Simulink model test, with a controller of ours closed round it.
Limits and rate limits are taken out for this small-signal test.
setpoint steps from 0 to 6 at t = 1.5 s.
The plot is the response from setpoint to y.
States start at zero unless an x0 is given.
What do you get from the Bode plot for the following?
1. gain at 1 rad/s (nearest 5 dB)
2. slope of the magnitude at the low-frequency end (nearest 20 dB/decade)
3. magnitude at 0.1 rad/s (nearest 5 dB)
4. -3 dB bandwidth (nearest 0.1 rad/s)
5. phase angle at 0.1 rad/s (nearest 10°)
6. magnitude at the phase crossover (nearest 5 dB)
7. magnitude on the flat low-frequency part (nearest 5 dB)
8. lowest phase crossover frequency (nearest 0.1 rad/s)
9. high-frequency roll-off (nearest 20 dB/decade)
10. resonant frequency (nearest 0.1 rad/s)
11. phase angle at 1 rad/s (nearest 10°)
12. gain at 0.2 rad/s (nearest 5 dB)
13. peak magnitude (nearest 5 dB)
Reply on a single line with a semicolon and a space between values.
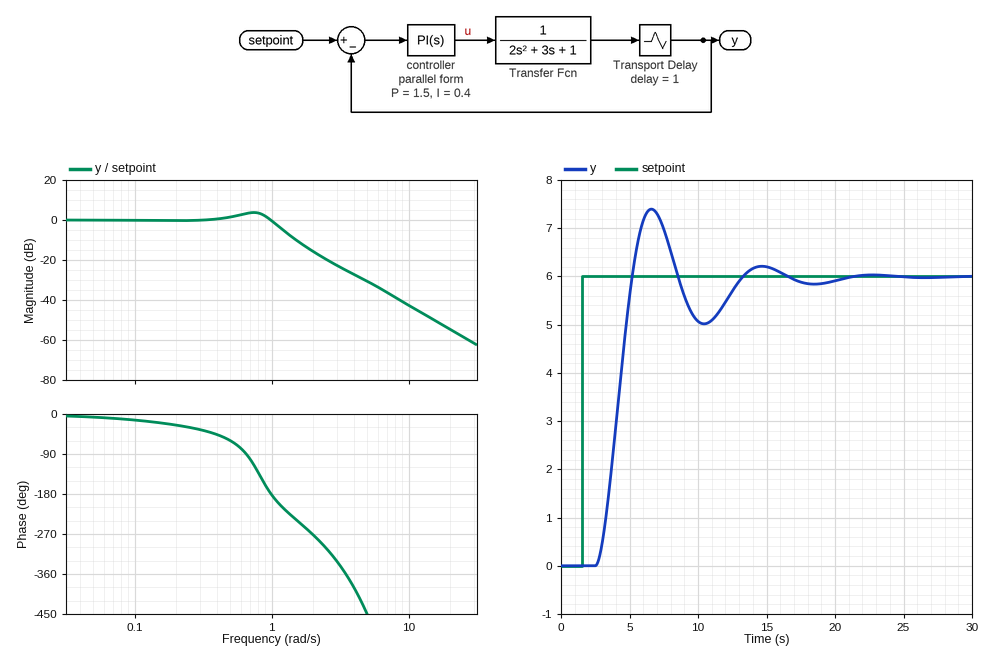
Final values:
0 dB; 0 dB/decade; 0 dB; 1.1 rad/s; -10°; 0 dB; 0 dB; 1.0 rad/s; -40 dB/decade; 0.7 rad/s; -180°; 0 dB; 5 dB
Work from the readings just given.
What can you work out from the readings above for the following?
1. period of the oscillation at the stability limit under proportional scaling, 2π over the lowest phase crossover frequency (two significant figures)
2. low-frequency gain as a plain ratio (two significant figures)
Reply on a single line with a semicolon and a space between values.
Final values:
6.3 s; 1.0
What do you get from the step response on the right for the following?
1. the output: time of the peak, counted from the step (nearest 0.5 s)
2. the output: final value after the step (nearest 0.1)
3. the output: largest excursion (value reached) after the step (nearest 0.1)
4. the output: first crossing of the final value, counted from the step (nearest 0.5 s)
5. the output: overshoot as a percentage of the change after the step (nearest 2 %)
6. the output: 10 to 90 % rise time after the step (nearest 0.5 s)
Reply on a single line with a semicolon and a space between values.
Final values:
5.0 s; 6.0; 7.4; 3.5 s; 24 %; 2.0 s
